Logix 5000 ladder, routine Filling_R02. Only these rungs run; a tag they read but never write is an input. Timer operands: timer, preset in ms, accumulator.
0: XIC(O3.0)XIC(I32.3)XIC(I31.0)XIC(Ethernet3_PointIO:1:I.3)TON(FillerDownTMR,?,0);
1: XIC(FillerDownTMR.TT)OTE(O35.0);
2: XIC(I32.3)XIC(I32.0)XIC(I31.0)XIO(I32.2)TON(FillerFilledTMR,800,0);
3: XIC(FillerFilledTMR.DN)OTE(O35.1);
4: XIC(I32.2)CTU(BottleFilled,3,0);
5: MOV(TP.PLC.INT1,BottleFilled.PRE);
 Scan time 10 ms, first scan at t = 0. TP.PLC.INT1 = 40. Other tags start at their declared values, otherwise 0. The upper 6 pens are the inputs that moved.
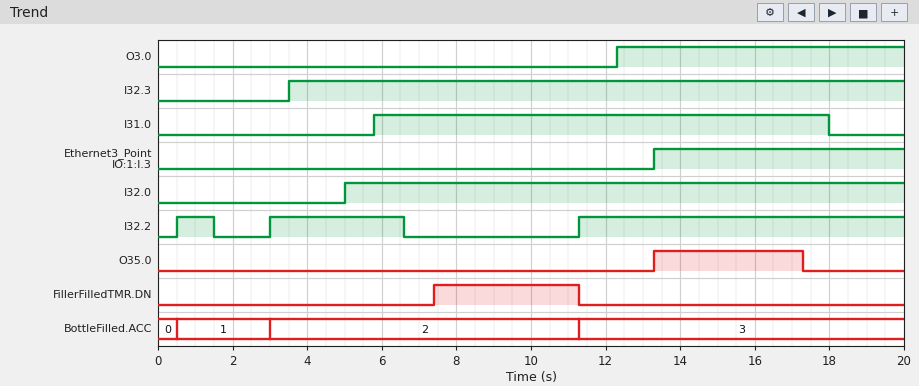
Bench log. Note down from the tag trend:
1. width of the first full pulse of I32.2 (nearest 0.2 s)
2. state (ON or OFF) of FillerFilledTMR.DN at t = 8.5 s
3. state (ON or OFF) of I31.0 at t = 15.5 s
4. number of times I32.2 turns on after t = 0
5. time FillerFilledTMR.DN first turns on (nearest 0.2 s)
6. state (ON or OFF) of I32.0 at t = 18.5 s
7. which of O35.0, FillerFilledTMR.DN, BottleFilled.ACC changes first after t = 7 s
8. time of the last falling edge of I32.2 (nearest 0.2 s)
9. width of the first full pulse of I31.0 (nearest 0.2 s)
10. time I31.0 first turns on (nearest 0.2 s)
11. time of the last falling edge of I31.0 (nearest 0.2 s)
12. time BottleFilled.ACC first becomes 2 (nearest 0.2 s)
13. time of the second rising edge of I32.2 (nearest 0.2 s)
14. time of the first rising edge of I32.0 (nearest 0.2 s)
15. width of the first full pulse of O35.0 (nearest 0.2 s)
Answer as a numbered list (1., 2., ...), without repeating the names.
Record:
1. 1.0 s
2. ON
3. ON
4. 3
5. 7.4 s
6. ON
7. FillerFilledTMR.DN
8. 6.6 s
9. 12.2 s
10. 5.8 s
11. 18.0 s
12. 3.0 s
13. 3.0 s
14. 5.0 s
15. 4.0 s
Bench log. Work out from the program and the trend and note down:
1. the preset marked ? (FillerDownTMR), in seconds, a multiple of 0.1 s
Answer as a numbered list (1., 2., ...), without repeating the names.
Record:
1. 4.0 s
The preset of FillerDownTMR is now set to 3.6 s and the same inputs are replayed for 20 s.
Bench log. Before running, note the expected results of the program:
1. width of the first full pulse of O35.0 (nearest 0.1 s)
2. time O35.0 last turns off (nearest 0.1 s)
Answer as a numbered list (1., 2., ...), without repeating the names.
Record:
1. 3.6 s
2. 16.9 s
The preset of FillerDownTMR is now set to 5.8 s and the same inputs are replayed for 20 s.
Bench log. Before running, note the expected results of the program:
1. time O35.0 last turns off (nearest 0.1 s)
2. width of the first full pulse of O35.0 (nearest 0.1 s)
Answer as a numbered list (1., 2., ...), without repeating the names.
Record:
1. 18.0 s
2. 4.7 s
